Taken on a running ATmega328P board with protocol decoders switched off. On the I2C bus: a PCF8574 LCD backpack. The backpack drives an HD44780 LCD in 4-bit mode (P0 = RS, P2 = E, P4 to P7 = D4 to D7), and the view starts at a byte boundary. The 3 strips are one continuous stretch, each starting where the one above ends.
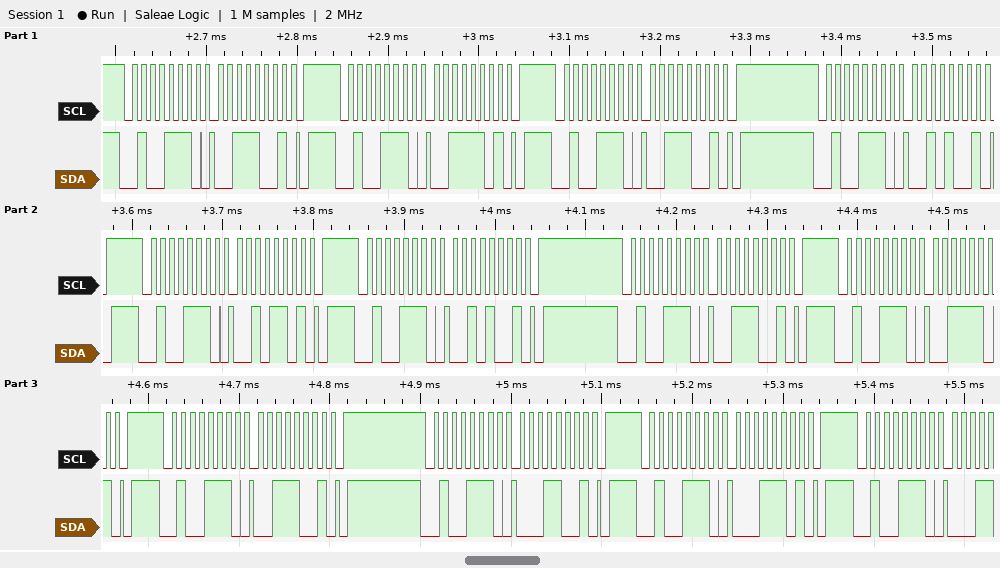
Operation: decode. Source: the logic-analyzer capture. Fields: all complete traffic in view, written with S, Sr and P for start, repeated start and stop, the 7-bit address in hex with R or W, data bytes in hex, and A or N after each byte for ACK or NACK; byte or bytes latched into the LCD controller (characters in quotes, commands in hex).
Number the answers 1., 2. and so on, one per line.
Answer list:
1. S 27W A 39 A P S 27W A 3D A P S 27W A 39 A P S 27W A 29 A P S 27W A 2D A P S 27W A 29 A P S 27W A 39 A P S 27W A 3D A P S 27W A 39 A P S 27W A 19 A P S 27W A 1D A P S 27W A
2. '2'
